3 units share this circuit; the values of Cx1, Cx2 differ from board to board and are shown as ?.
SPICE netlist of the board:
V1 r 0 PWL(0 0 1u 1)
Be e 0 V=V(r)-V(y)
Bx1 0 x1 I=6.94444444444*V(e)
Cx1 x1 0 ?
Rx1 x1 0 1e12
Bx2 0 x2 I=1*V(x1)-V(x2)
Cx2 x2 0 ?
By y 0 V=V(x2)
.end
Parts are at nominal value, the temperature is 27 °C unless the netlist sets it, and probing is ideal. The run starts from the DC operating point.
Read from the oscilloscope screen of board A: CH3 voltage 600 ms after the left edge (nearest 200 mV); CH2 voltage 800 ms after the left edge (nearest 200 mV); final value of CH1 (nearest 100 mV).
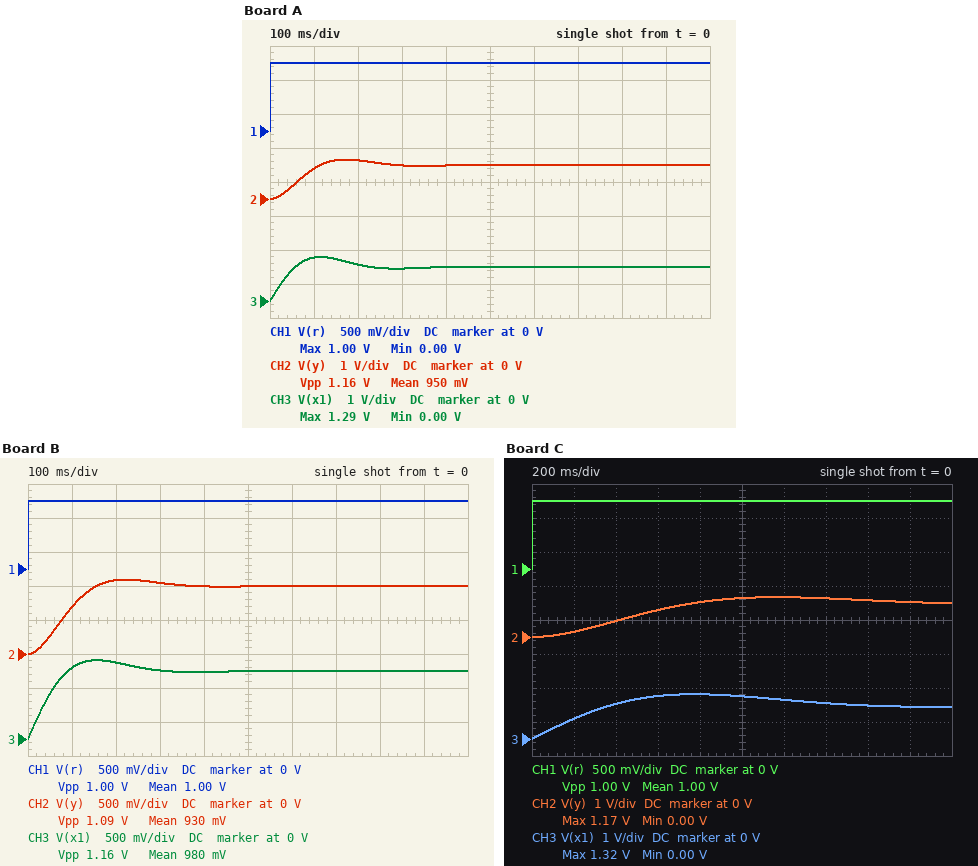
1.0 V
1.0 V
1.0 V
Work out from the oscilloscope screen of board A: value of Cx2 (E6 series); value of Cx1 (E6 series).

47 mF
330 mF
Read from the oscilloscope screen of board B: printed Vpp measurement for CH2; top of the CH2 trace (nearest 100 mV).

1.09 V
1.1 V
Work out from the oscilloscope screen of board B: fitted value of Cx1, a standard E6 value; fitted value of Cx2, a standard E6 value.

470 mF
47 mF
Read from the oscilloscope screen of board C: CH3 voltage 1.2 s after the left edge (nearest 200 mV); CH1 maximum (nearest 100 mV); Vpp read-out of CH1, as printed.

1.2 V
1.0 V
1.00 V
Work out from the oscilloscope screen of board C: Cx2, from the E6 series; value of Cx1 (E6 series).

330 mF
2.2 F
